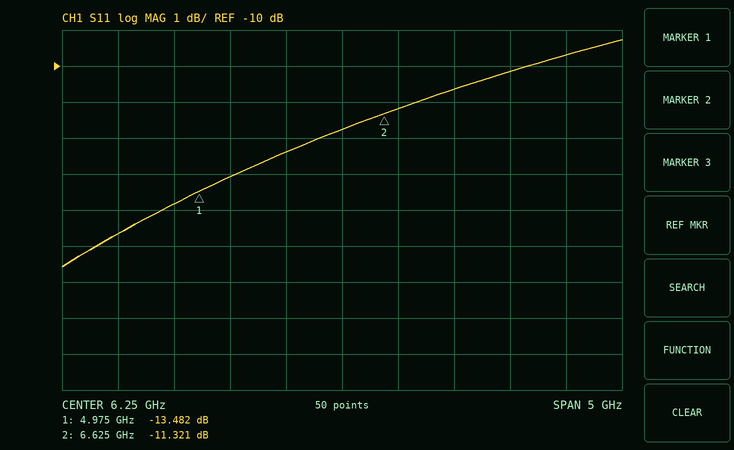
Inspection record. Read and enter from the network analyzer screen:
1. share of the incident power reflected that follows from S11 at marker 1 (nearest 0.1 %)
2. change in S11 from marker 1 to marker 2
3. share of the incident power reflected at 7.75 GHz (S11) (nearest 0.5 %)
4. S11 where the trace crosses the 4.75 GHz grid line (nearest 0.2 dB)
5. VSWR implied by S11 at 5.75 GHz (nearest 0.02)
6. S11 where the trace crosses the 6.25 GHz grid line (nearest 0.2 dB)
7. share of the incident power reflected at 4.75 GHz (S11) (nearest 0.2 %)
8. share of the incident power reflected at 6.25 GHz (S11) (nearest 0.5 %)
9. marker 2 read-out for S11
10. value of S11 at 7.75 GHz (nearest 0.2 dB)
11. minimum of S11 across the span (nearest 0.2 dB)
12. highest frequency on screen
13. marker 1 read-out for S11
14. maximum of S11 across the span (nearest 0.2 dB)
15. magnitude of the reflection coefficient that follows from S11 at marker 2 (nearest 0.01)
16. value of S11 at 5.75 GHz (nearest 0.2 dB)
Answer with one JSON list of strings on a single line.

["4.5 %", "2.161 dB", "9.5 %", "-13.8 dB", "1.64", "-11.8 dB", "4.2 %", "6.5 %", "-11.321 dB", "-10.2 dB", "-15.6 dB", "8.75 GHz", "-13.482 dB", "-9.2 dB", "0.27", "-12.4 dB"]
